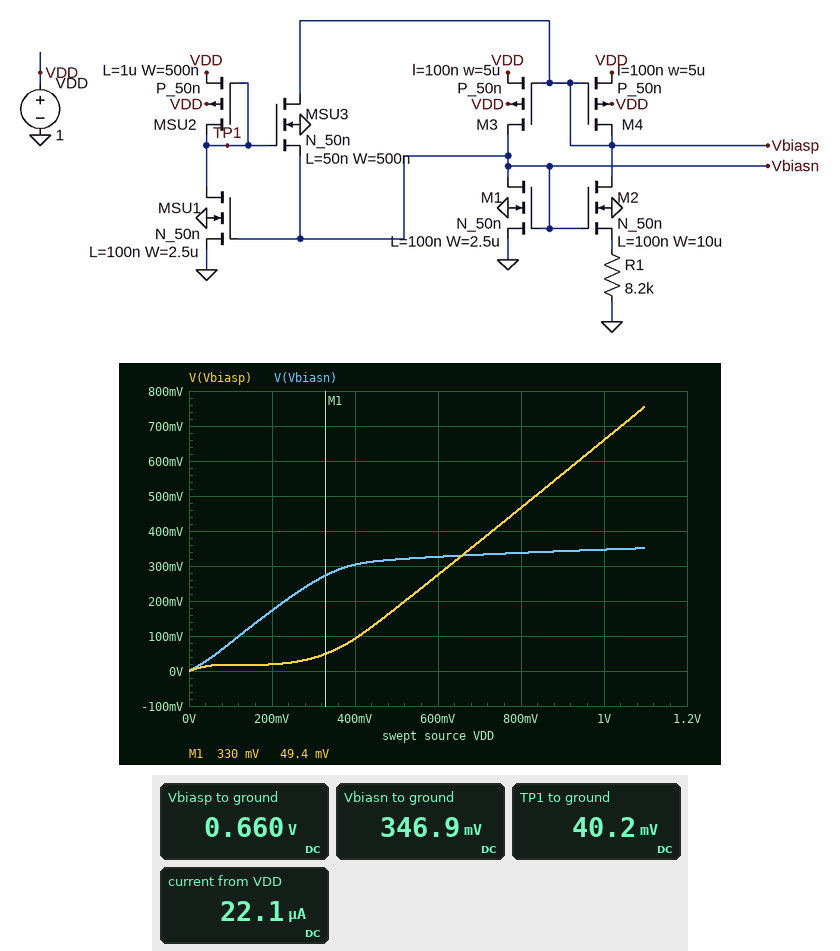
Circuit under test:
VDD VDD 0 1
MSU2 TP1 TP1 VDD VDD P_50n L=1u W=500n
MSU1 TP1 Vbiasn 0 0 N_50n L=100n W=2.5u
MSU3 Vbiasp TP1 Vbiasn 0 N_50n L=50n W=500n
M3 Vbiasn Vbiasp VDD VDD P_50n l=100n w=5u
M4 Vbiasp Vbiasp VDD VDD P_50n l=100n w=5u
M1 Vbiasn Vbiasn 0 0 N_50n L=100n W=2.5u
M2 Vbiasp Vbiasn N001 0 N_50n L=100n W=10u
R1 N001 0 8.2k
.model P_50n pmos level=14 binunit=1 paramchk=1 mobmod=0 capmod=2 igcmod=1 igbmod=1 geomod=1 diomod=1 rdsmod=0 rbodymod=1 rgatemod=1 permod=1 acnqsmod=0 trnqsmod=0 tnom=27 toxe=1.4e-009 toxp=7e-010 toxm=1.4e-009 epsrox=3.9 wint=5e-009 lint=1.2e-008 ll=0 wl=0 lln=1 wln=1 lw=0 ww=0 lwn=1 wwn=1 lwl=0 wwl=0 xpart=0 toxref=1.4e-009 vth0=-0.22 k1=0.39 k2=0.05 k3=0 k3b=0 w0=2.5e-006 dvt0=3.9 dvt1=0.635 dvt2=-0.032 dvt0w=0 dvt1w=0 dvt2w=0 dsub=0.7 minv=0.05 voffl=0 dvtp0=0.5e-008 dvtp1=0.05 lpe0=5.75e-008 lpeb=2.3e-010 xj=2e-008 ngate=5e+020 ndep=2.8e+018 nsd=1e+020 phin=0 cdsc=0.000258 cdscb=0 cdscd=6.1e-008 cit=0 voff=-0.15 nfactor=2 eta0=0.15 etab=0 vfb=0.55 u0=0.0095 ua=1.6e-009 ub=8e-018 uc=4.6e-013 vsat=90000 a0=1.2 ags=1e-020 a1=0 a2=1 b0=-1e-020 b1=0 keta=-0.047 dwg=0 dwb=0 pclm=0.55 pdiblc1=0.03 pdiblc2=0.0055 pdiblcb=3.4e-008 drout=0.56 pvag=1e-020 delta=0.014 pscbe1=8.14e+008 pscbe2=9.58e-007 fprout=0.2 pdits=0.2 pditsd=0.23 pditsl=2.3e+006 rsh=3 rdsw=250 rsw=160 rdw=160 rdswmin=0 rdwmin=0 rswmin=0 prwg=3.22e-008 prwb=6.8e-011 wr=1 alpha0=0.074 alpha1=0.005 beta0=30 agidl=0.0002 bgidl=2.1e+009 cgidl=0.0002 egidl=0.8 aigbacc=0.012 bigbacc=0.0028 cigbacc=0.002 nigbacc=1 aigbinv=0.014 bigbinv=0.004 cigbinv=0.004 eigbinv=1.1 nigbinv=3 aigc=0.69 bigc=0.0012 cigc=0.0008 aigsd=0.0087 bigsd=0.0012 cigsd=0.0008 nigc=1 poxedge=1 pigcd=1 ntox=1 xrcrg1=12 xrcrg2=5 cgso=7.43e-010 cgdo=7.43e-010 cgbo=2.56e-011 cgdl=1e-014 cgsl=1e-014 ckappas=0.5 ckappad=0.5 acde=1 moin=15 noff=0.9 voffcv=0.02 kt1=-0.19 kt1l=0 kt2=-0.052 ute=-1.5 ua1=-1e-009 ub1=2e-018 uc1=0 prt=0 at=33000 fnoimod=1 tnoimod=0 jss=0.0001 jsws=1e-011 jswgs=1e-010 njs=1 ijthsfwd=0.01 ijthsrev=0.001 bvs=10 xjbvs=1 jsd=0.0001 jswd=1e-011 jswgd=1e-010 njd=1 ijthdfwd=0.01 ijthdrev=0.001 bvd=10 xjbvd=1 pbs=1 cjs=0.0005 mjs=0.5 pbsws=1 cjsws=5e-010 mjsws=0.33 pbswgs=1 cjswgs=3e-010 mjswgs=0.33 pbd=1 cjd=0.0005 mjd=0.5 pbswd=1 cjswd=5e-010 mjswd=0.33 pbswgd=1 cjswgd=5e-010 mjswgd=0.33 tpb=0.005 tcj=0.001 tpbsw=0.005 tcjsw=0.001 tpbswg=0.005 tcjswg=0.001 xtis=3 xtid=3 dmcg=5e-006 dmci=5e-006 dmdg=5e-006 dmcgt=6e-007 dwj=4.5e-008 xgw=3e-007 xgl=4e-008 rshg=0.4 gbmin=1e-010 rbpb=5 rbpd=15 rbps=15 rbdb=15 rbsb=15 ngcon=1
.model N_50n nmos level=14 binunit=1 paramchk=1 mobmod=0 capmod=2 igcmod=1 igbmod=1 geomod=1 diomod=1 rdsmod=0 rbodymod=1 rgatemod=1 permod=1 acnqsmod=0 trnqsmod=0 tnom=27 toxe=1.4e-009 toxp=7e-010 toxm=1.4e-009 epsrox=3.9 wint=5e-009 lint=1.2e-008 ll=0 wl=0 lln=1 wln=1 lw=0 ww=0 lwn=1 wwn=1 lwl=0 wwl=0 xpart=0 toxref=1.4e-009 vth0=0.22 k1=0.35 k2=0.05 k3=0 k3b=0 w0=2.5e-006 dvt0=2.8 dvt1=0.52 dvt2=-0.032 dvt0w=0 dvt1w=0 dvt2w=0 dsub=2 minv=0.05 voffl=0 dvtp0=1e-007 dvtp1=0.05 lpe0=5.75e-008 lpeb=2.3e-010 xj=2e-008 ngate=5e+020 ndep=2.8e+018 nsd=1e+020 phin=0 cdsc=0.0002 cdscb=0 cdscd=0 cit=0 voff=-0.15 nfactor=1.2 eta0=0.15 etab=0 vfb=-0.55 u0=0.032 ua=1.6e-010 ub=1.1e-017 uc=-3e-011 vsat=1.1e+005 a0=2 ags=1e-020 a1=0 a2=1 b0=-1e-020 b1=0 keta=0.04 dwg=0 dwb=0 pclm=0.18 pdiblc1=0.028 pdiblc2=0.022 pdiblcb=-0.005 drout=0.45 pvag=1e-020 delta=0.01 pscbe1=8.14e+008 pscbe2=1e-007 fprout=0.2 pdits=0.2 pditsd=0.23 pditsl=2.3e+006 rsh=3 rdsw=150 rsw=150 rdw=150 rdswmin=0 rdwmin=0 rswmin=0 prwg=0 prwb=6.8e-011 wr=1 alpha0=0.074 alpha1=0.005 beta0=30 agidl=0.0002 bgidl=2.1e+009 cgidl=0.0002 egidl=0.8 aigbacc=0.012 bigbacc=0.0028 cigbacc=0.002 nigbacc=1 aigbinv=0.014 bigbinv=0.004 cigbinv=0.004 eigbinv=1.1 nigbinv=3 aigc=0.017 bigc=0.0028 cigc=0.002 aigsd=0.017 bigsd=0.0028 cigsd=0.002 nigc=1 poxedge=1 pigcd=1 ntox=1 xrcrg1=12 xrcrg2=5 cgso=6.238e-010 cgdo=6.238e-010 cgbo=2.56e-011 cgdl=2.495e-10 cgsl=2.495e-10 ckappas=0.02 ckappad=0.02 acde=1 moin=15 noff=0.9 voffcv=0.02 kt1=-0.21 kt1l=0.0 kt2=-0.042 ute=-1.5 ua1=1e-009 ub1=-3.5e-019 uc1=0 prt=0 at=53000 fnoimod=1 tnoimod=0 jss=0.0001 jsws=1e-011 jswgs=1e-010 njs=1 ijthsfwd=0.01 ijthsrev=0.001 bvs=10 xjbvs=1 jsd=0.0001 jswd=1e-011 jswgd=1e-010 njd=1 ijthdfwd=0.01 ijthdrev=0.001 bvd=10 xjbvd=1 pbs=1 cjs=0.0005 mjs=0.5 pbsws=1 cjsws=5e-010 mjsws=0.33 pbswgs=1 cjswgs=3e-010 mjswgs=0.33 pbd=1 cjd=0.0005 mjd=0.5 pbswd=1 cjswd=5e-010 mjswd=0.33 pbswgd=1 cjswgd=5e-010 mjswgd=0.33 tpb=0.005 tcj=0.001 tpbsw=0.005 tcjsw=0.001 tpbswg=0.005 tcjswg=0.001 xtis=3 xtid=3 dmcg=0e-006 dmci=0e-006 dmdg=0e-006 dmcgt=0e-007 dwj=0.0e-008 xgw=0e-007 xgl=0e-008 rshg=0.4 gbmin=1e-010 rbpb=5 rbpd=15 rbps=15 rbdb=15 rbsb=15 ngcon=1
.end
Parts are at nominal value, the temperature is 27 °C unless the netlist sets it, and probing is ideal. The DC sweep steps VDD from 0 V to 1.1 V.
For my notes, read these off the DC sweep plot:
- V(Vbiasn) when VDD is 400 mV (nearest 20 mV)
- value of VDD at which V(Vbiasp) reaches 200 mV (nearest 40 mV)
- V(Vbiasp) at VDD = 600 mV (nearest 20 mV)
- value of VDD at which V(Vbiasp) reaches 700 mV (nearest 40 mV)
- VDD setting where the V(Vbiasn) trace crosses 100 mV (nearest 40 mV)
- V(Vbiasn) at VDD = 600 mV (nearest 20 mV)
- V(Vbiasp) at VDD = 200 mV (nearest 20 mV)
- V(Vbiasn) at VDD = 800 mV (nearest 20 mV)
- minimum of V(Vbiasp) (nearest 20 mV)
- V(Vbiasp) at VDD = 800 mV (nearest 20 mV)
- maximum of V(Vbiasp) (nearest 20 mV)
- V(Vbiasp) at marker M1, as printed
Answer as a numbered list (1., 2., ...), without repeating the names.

1. 300 mV
2. 520 mV
3. 280 mV
4. 1.04 V
5. 120 mV
6. 320 mV
7. 20 mV
8. 340 mV
9. 0 V
10. 460 mV
11. 760 mV
12. 49.4 mV
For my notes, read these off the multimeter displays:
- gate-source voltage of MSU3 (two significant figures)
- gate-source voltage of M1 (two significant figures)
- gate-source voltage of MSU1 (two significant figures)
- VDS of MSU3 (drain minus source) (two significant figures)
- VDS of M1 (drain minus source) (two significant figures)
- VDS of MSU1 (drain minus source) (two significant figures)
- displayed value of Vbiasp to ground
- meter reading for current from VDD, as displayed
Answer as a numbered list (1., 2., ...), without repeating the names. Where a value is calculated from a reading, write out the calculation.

1. 40.2 mV - 346.9 mV = -310 mV
2. 346.9 mV = 350 mV
3. 346.9 mV = 350 mV
4. 660 mV - 346.9 mV = 310 mV
5. 346.9 mV = 350 mV
6. 40.2 mV = 40 mV
7. 0.660 V
8. 22.1 µA
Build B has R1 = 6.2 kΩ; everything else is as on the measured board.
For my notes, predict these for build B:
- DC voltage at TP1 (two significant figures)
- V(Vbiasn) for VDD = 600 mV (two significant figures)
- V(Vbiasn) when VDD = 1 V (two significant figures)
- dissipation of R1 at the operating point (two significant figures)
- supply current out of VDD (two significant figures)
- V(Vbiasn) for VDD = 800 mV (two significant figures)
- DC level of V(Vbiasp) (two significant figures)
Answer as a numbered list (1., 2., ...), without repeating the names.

1. 29 mV
2. 340 mV
3. 360 mV
4. 710 nW
5. 28 µA
6. 350 mV
7. 640 mV
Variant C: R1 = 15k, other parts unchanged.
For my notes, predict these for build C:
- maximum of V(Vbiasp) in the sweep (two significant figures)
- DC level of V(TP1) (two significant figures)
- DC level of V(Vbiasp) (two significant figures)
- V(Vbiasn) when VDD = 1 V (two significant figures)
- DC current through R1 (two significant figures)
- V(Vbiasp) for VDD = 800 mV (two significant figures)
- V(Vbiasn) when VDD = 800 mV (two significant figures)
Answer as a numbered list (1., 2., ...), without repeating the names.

1. 790 mV
2. 160 mV
3. 690 mV
4. 320 mV
5. 4.3 µA
6. 500 mV
7. 310 mV
